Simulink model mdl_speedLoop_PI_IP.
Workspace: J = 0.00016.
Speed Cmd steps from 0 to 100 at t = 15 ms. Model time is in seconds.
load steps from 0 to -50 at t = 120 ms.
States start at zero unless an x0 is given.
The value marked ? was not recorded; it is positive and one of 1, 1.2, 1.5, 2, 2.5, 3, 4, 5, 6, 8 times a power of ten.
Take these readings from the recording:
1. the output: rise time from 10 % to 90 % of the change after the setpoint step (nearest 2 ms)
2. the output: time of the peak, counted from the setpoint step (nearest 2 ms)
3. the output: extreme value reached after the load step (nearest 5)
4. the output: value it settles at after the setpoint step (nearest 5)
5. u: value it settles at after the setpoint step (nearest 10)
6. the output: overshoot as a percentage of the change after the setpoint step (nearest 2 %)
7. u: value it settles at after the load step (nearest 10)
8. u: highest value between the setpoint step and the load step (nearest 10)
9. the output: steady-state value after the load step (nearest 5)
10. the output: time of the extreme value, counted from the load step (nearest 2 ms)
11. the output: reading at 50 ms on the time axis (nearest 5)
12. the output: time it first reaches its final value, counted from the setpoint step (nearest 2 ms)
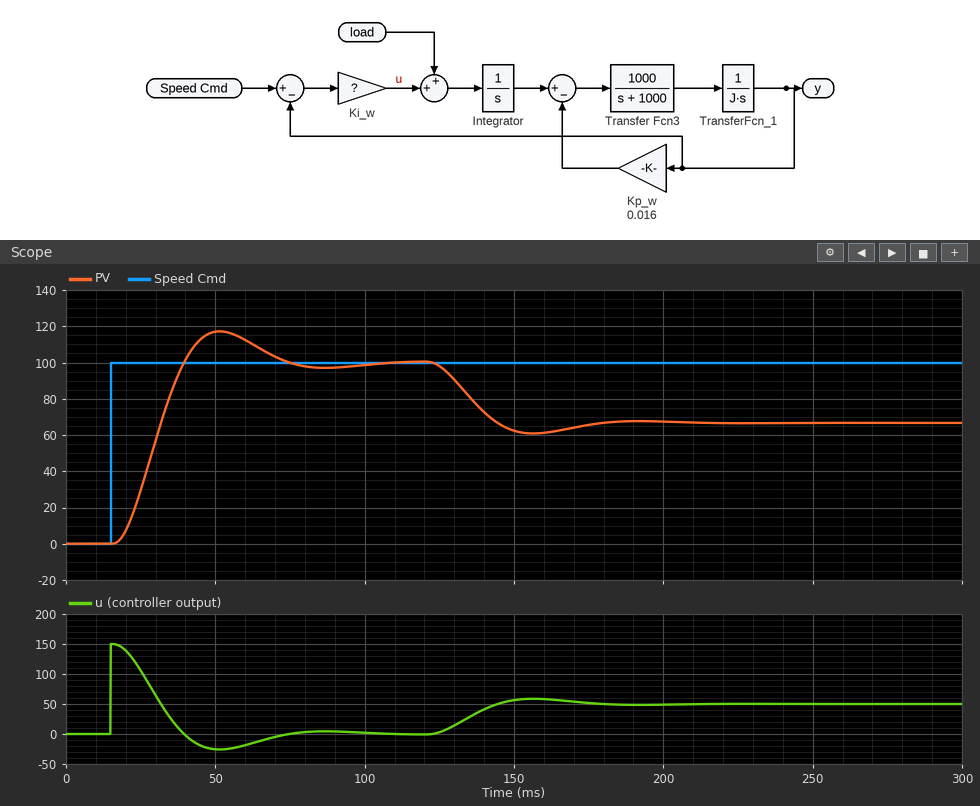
16 ms
36 ms
60
100
0
18 %
50
150
65
36 ms
115
24 ms
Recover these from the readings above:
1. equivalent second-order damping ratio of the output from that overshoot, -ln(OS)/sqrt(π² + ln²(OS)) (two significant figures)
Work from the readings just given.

0.48
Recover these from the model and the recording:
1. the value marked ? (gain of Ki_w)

1.5
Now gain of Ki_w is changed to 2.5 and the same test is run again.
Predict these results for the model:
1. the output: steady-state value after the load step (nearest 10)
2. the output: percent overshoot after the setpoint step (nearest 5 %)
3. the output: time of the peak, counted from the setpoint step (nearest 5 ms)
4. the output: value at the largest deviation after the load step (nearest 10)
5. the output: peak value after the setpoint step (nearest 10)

80
30 %
25 ms
70
130
